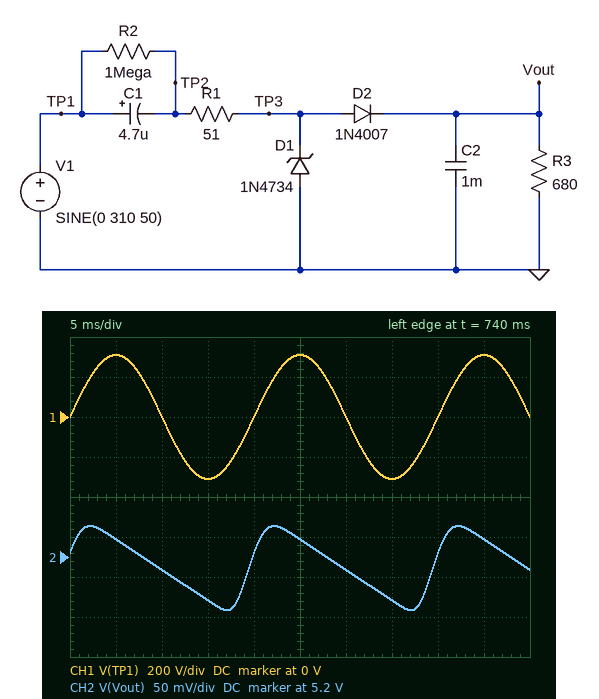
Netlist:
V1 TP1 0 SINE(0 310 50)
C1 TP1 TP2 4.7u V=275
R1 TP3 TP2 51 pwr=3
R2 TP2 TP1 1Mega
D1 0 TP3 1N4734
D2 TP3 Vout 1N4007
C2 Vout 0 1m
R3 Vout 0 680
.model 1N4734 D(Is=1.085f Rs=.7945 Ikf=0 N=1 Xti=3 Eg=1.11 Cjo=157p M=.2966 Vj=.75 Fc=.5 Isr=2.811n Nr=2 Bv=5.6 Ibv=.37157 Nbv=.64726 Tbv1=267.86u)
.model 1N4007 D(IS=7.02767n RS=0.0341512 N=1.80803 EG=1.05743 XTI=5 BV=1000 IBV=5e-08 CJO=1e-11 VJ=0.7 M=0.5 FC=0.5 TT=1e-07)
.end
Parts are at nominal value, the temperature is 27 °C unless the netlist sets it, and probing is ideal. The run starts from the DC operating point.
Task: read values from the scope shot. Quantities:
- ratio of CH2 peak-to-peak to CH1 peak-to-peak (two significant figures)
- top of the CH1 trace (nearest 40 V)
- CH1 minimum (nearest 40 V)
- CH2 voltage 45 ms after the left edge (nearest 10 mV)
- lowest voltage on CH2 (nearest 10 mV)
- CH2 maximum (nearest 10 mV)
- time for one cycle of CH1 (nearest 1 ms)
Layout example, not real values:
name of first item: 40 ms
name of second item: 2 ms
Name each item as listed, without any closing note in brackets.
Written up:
ratio of CH2 peak-to-peak to CH1 peak-to-peak: 0.00017
top of the CH1 trace: 320 V
CH1 minimum: -320 V
CH2 voltage 45 ms after the left edge: 5.22 V
lowest voltage on CH2: 5.13 V
CH2 maximum: 5.24 V
time for one cycle of CH1: 20 ms
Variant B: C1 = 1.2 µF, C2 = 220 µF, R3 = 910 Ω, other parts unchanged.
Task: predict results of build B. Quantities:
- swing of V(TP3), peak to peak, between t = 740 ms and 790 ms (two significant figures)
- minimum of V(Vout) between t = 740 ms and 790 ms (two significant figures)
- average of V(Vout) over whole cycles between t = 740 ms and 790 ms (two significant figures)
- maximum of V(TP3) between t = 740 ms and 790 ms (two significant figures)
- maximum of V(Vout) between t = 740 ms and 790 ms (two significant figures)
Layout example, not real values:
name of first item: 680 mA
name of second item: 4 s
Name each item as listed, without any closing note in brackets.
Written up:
swing of V(TP3), peak to peak, between t = 740 ms and 790 ms: 6.6 V
minimum of V(Vout) between t = 740 ms and 790 ms: 4.7 V
average of V(Vout) over whole cycles between t = 740 ms and 790 ms: 4.9 V
maximum of V(TP3) between t = 740 ms and 790 ms: 5.7 V
maximum of V(Vout) between t = 740 ms and 790 ms: 5.0 V
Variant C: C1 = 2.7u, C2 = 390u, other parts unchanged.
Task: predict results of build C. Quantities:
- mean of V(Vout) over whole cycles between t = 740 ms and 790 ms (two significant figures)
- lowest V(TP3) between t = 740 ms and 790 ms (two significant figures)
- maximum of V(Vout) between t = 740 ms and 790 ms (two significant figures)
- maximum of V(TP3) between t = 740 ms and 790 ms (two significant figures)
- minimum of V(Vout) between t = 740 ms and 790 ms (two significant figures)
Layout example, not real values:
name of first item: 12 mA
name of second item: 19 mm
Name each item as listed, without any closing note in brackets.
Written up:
mean of V(Vout) over whole cycles between t = 740 ms and 790 ms: 5.0 V
lowest V(TP3) between t = 740 ms and 790 ms: -1.1 V
maximum of V(Vout) between t = 740 ms and 790 ms: 5.1 V
maximum of V(TP3) between t = 740 ms and 790 ms: 5.8 V
minimum of V(Vout) between t = 740 ms and 790 ms: 4.9 V
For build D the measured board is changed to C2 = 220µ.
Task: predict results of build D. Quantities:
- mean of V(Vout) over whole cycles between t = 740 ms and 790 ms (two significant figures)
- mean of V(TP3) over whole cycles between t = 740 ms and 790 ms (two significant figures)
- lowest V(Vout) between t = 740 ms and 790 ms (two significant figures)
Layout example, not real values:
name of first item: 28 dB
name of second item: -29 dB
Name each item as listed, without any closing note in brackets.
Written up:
mean of V(Vout) over whole cycles between t = 740 ms and 790 ms: 5.1 V
mean of V(TP3) over whole cycles between t = 740 ms and 790 ms: 2.4 V
lowest V(Vout) between t = 740 ms and 790 ms: 4.8 V
